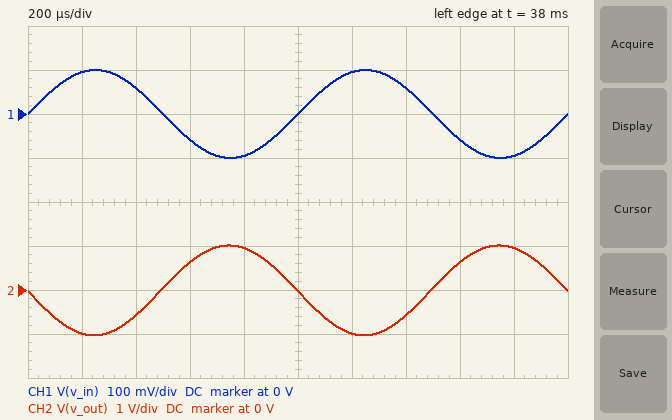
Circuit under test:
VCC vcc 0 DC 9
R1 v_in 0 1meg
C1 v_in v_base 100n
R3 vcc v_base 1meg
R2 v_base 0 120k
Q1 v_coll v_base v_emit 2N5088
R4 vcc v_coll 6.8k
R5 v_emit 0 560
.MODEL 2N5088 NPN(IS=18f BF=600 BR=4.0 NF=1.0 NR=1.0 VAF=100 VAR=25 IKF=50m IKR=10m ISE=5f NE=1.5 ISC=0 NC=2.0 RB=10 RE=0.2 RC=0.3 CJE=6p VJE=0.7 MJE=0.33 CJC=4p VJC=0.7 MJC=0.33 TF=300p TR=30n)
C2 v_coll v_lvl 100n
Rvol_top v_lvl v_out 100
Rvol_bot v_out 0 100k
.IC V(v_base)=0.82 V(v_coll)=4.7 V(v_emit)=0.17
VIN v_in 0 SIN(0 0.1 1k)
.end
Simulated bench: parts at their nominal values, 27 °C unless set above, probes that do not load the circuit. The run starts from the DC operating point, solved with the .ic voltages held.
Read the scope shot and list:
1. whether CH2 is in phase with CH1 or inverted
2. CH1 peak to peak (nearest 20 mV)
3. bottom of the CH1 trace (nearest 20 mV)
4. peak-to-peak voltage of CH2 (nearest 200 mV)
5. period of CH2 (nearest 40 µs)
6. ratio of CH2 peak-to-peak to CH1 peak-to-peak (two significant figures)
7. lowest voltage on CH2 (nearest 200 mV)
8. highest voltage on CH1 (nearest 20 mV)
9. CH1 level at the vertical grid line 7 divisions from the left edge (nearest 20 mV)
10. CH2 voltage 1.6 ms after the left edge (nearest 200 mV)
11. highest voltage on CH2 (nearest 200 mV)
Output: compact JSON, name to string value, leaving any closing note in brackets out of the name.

{"whether CH2 is in phase with CH1 or inverted": "inverted", "CH1 peak to peak": "200 mV", "bottom of the CH1 trace": "-100 mV", "peak-to-peak voltage of CH2": "2.0 V", "period of CH2": "1.00 ms", "ratio of CH2 peak-to-peak to CH1 peak-to-peak": "10", "lowest voltage on CH2": "-1.0 V", "highest voltage on CH1": "100 mV", "CH1 level at the vertical grid line 7 divisions from the left edge": "60 mV", "CH2 voltage 1.6 ms after the left edge": "600 mV", "highest voltage on CH2": "1.0 V"}
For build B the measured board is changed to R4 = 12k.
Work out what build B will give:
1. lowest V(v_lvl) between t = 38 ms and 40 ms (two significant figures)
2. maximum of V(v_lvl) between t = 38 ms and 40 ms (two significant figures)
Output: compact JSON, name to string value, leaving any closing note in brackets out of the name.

{"lowest V(v_lvl) between t = 38 ms and 40 ms": "-1.8 V", "maximum of V(v_lvl) between t = 38 ms and 40 ms": "1.6 V"}
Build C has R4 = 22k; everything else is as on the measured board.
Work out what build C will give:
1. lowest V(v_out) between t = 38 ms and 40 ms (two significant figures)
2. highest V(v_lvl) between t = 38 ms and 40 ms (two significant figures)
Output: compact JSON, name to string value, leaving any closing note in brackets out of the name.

{"lowest V(v_out) between t = 38 ms and 40 ms": "-2.5 V", "highest V(v_lvl) between t = 38 ms and 40 ms": "2.6 V"}
